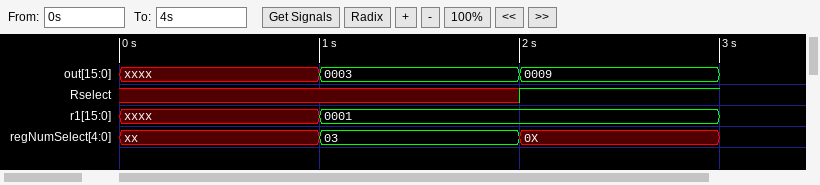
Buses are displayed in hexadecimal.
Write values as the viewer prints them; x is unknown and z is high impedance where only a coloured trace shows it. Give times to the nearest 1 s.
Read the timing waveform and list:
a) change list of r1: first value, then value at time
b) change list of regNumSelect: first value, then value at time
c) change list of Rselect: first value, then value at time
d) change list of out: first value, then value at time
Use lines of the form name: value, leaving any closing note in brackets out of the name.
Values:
change list of r1: first value, then value at time: xxxx, 0001 at 1 s
change list of regNumSelect: first value, then value at time: xx, 03 at 1 s, 0X at 2 s
change list of Rselect: first value, then value at time: x, 1 at 2 s
change list of out: first value, then value at time: xxxx, 0003 at 1 s, 0009 at 2 s
